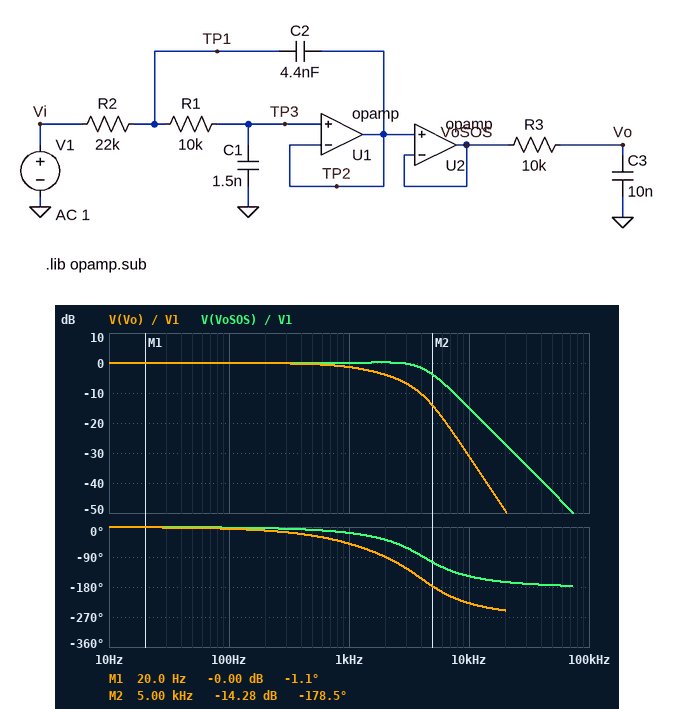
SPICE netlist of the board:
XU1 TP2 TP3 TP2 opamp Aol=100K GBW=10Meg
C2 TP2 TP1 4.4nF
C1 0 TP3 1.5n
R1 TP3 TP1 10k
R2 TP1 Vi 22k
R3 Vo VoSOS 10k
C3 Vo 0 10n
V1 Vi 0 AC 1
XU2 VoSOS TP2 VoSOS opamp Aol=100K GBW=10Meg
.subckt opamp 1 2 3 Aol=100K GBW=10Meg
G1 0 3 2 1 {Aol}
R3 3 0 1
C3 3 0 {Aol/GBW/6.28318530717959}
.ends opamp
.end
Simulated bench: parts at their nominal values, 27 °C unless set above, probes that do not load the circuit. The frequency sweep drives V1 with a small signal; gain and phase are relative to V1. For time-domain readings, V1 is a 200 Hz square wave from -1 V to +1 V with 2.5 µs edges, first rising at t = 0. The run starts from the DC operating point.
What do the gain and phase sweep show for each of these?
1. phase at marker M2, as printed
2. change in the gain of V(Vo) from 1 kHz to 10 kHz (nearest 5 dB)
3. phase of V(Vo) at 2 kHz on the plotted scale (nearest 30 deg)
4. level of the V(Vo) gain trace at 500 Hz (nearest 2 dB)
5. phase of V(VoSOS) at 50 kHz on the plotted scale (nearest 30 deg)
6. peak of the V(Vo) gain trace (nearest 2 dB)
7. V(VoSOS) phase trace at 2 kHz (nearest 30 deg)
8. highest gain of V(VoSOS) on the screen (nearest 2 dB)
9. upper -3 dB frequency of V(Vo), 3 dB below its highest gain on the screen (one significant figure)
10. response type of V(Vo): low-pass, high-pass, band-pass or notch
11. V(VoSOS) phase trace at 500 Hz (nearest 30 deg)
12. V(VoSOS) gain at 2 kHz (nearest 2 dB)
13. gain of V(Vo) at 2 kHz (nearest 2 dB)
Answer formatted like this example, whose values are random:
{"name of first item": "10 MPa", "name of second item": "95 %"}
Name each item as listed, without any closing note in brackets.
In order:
{"phase at marker M2, as printed": "-178.5 deg", "change in the gain of V(Vo) from 1 kHz to 10 kHz": "-30 dB", "phase of V(Vo) at 2 kHz on the plotted scale": "-90 deg", "level of the V(Vo) gain trace at 500 Hz": "0 dB", "phase of V(VoSOS) at 50 kHz on the plotted scale": "-180 deg", "peak of the V(Vo) gain trace": "0 dB", "V(VoSOS) phase trace at 2 kHz": "-30 deg", "highest gain of V(VoSOS) on the screen": "0 dB", "upper -3 dB frequency of V(Vo), 3 dB below its highest gain on the screen": "2 kHz", "response type of V(Vo): low-pass, high-pass, band-pass or notch": "low-pass", "V(VoSOS) phase trace at 500 Hz": "0 deg", "V(VoSOS) gain at 2 kHz": "0 dB", "gain of V(Vo) at 2 kHz": "-4 dB"}
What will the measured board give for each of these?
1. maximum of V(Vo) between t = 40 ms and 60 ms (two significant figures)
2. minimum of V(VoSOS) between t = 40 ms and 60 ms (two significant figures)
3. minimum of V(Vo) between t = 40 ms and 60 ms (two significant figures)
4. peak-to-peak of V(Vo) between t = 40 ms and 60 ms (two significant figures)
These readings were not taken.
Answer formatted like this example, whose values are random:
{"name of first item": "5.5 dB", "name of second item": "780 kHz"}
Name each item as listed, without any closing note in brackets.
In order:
{"maximum of V(Vo) between t = 40 ms and 60 ms": "1.0 V", "minimum of V(VoSOS) between t = 40 ms and 60 ms": "-1.2 V", "minimum of V(Vo) between t = 40 ms and 60 ms": "-1.0 V", "peak-to-peak of V(Vo) between t = 40 ms and 60 ms": "2.0 V"}
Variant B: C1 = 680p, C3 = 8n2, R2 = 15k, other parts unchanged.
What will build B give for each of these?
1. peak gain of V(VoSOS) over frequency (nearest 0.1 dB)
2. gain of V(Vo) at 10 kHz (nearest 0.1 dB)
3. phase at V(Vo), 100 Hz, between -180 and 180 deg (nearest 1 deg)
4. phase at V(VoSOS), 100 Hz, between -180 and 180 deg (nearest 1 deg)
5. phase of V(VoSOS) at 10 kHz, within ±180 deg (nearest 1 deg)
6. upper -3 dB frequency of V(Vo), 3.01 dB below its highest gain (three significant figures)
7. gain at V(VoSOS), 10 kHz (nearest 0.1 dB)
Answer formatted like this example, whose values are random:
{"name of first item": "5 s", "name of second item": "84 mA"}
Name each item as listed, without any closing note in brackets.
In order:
{"peak gain of V(VoSOS) over frequency": "2.7 dB", "gain of V(Vo) at 10 kHz": "-16.8 dB", "phase at V(Vo), 100 Hz, between -180 and 180 deg": "-4 deg", "phase at V(VoSOS), 100 Hz, between -180 and 180 deg": "-1 deg", "phase of V(VoSOS) at 10 kHz, within ±180 deg": "-126 deg", "upper -3 dB frequency of V(Vo), 3.01 dB below its highest gain": "2.16 kHz", "gain at V(VoSOS), 10 kHz": "-2.4 dB"}
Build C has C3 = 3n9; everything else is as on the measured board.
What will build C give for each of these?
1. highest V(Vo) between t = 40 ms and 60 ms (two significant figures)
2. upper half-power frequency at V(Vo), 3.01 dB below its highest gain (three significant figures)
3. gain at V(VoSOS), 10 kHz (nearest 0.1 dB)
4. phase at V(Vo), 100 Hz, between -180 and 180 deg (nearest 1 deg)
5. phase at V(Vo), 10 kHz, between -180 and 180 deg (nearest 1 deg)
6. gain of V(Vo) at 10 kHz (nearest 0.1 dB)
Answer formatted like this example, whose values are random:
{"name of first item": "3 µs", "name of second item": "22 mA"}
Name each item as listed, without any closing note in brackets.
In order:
{"highest V(Vo) between t = 40 ms and 60 ms": "1.1 V", "upper half-power frequency at V(Vo), 3.01 dB below its highest gain": "3.42 kHz", "gain at V(VoSOS), 10 kHz": "-15.0 dB", "phase at V(Vo), 100 Hz, between -180 and 180 deg": "-3 deg", "phase at V(Vo), 10 kHz, between -180 and 180 deg": "145 deg", "gain of V(Vo) at 10 kHz": "-23.4 dB"}
